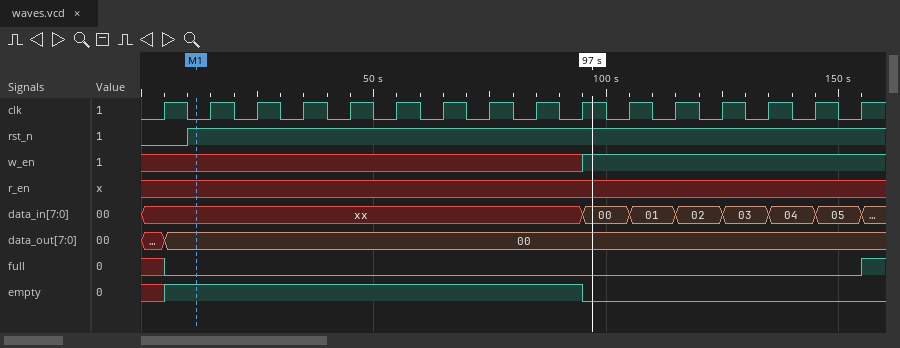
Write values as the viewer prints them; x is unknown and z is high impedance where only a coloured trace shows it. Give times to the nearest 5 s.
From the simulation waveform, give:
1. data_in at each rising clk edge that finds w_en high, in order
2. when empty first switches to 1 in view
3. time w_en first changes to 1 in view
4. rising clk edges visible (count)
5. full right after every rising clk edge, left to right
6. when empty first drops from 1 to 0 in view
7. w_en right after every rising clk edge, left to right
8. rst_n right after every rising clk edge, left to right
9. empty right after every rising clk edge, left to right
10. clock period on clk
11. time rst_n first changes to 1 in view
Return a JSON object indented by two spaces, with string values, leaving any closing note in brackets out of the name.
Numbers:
{
  "data_in at each rising clk edge that finds w_en high, in order": "00, 01, 02, 03, 04, 05",
  "when empty first switches to 1 in view": "5 s",
  "time w_en first changes to 1 in view": "95 s",
  "rising clk edges visible": "16",
  "full right after every rising clk edge, left to right": "0 0 0 0 0 0 0 0 0 0 0 0 0 0 0 1",
  "when empty first drops from 1 to 0 in view": "95 s",
  "w_en right after every rising clk edge, left to right": "x x x x x x x x x 1 1 1 1 1 1 1",
  "rst_n right after every rising clk edge, left to right": "0 1 1 1 1 1 1 1 1 1 1 1 1 1 1 1",
  "empty right after every rising clk edge, left to right": "1 1 1 1 1 1 1 1 1 0 0 0 0 0 0 0",
  "clock period on clk": "10 s",
  "time rst_n first changes to 1 in view": "10 s"
}
